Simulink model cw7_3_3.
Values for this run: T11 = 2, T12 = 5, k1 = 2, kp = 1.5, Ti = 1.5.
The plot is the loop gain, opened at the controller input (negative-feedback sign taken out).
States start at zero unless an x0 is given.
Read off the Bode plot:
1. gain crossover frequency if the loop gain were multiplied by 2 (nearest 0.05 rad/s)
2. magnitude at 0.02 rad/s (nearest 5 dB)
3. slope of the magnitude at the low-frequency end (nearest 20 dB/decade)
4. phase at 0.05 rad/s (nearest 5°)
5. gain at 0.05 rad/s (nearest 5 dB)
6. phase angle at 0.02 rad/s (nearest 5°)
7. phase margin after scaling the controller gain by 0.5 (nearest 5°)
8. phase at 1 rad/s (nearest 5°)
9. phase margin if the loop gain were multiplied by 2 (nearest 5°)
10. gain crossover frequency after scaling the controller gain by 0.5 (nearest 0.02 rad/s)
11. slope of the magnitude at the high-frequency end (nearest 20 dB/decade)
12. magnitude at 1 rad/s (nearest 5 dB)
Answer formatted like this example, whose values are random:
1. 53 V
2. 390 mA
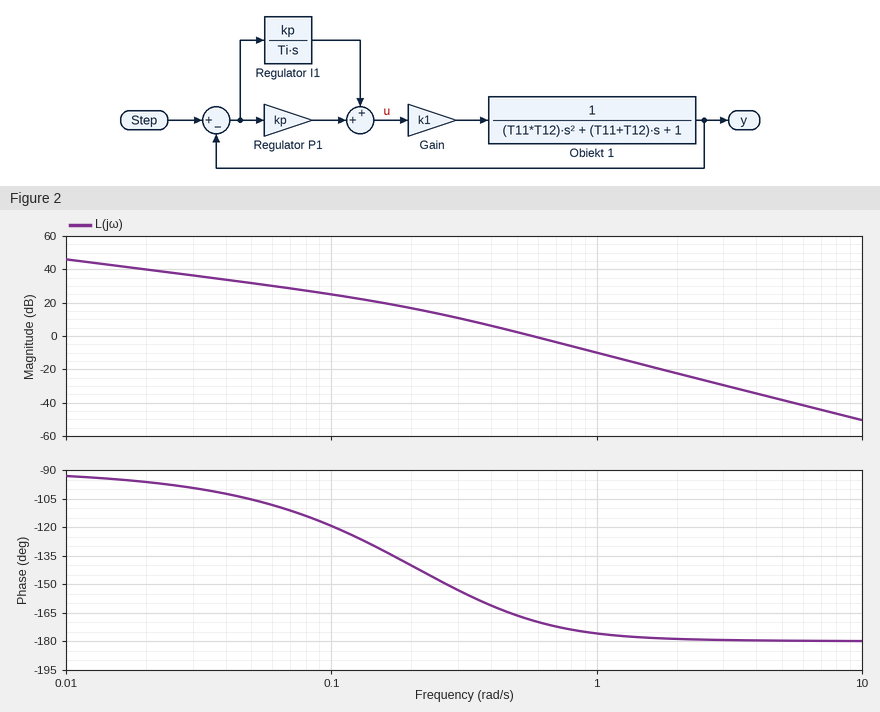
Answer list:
1. 0.80 rad/s
2. 40 dB
3. -20 dB/decade
4. -105°
5. 30 dB
6. -95°
7. 20°
8. -175°
9. 5°
10. 0.40 rad/s
11. -40 dB/decade
12. -10 dB
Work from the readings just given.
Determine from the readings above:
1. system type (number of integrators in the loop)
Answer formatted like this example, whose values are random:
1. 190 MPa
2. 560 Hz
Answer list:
1. 1
